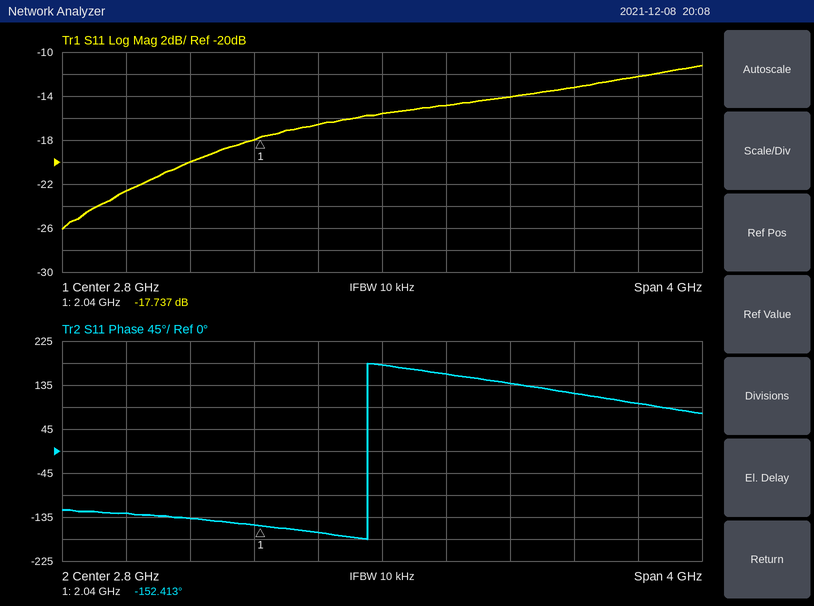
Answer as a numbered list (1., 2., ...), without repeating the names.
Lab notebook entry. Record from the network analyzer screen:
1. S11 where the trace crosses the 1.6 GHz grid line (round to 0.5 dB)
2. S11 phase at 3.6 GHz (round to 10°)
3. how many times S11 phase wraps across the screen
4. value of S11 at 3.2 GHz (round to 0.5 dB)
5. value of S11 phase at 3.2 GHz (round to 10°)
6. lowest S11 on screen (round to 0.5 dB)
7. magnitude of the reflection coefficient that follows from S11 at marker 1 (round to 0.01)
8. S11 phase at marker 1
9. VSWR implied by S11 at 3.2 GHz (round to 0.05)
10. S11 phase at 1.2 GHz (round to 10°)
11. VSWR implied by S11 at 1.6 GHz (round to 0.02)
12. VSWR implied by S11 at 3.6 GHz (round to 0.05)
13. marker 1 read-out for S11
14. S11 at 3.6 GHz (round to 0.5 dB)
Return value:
1. -20.0 dB
2. 140°
3. 1
4. -15.0 dB
5. 160°
6. -26.0 dB
7. 0.13
8. -152.413°
9. 1.45
10. -130°
11. 1.22
12. 1.50
13. -17.737 dB
14. -14.0 dB
